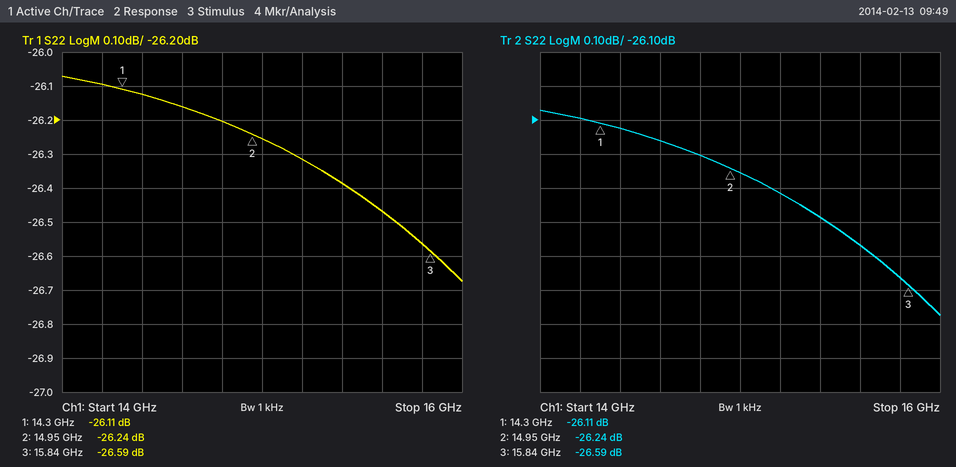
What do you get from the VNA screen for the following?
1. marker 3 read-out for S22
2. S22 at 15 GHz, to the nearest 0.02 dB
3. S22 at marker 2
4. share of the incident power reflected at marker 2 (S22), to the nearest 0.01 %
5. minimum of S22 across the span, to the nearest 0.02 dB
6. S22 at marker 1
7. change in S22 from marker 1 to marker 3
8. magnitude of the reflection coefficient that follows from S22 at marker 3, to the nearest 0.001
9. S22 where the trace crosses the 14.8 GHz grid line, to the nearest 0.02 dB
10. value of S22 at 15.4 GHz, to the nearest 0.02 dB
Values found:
-26.59 dB
-26.26 dB
-26.24 dB
0.24 %
-26.68 dB
-26.11 dB
-0.48 dB
0.047
-26.20 dB
-26.38 dB
